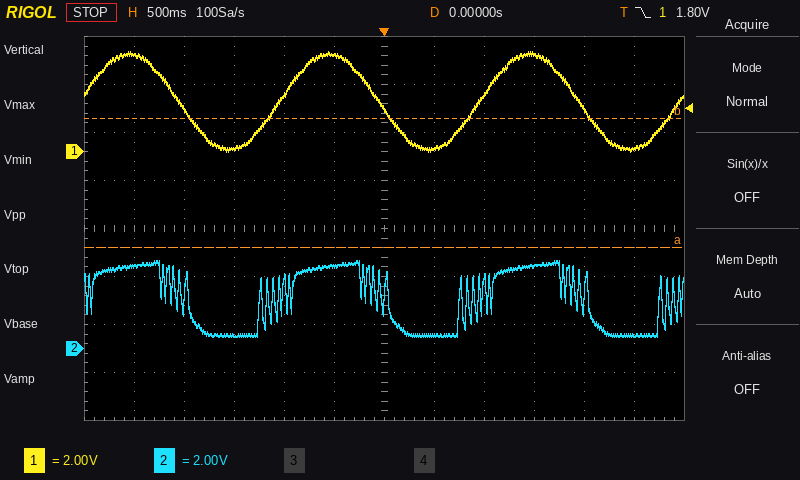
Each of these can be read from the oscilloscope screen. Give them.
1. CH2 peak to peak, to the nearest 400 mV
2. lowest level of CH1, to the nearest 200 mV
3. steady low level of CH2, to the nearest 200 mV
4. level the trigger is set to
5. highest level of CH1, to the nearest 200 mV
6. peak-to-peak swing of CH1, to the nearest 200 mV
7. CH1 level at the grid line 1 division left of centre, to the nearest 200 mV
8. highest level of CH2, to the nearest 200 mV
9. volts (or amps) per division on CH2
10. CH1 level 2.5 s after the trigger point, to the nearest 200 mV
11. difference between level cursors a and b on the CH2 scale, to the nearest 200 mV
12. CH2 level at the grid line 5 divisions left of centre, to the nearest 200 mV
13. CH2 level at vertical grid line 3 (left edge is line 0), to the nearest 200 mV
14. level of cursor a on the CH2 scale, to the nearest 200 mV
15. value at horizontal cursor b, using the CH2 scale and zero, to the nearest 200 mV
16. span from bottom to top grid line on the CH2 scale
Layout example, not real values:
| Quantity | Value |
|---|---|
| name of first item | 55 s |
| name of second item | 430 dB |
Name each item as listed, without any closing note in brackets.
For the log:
| Quantity | Value |
|---|---|
| CH2 peak to peak, to the nearest 400 mV | 3.2 V |
| lowest level of CH1, to the nearest 200 mV | 0.0 V |
| steady low level of CH2, to the nearest 200 mV | 600 mV |
| level the trigger is set to | 1.80 V |
| highest level of CH1, to the nearest 200 mV | 4.2 V |
| peak-to-peak swing of CH1, to the nearest 200 mV | 4.2 V |
| CH1 level at the grid line 1 division left of centre, to the nearest 200 mV | 4.0 V |
| highest level of CH2, to the nearest 200 mV | 3.6 V |
| volts (or amps) per division on CH2 | 2 V |
| CH1 level 2.5 s after the trigger point, to the nearest 200 mV | 200 mV |
| difference between level cursors a and b on the CH2 scale, to the nearest 200 mV | 5.4 V |
| CH2 level at the grid line 5 divisions left of centre, to the nearest 200 mV | 3.4 V |
| CH2 level at vertical grid line 3 (left edge is line 0), to the nearest 200 mV | 600 mV |
| level of cursor a on the CH2 scale, to the nearest 200 mV | 4.2 V |
| value at horizontal cursor b, using the CH2 scale and zero, to the nearest 200 mV | 9.6 V |
| span from bottom to top grid line on the CH2 scale | 16 V |
